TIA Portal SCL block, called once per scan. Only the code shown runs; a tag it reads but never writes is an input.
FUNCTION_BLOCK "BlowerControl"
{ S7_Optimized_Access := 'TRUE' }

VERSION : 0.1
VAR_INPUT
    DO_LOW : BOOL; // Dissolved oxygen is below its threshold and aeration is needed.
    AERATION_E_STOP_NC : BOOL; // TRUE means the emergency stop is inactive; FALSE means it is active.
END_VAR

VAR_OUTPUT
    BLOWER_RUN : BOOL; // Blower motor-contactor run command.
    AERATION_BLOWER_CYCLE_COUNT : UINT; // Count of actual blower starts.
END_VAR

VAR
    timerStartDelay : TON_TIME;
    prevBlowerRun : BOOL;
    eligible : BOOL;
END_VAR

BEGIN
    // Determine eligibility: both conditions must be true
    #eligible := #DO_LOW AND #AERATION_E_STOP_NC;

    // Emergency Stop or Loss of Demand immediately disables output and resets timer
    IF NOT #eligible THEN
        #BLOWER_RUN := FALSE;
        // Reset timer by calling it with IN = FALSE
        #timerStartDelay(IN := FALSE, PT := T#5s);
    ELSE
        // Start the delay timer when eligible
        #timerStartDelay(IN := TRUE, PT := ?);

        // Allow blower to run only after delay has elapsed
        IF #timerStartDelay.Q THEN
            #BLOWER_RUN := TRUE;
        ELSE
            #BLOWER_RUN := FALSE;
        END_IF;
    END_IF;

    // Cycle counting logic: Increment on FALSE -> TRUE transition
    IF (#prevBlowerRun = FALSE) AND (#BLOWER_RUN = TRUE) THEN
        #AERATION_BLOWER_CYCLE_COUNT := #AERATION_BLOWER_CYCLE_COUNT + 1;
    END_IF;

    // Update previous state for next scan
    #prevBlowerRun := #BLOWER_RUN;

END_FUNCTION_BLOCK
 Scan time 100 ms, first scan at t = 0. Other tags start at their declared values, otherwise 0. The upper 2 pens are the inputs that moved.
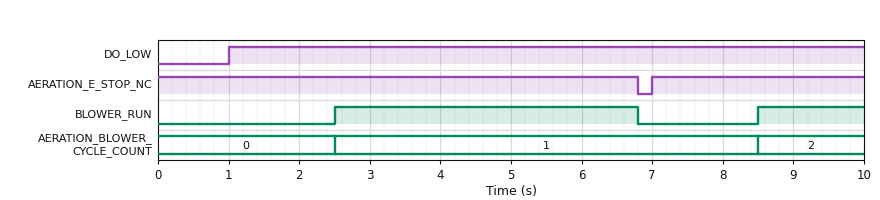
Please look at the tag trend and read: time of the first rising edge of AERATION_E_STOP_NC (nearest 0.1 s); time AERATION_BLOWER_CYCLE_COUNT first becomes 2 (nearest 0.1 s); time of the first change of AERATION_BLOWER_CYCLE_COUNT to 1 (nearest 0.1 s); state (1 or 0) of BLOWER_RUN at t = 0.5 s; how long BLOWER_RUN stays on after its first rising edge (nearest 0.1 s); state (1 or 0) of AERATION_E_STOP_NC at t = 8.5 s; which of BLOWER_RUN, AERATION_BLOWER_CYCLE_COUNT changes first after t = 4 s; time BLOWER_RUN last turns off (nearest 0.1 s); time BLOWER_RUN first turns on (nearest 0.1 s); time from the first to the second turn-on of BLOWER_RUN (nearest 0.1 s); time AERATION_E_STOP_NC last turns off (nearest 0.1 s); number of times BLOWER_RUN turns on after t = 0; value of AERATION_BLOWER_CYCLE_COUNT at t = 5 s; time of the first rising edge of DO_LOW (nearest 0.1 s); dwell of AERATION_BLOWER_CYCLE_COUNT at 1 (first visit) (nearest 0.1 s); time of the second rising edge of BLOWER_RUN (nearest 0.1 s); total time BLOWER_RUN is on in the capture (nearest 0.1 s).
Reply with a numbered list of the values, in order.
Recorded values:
1. 7.0 s
2. 8.5 s
3. 2.5 s
4. 0
5. 4.3 s
6. 1
7. BLOWER_RUN
8. 6.8 s
9. 2.5 s
10. 6.0 s
11. 6.8 s
12. 2
13. 1
14. 1.0 s
15. 6.0 s
16. 8.5 s
17. 5.8 s
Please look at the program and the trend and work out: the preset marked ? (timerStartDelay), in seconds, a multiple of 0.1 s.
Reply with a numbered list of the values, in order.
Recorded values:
1. 1.5 s
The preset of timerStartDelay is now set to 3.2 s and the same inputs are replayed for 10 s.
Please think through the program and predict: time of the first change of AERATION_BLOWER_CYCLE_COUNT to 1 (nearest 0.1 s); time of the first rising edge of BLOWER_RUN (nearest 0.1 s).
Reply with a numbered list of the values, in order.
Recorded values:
1. 4.2 s
2. 4.2 s
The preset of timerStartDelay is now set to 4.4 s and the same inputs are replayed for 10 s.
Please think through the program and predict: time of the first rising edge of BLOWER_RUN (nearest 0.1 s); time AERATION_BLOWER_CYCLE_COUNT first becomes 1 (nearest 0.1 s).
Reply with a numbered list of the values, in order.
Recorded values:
1. 5.4 s
2. 5.4 s
